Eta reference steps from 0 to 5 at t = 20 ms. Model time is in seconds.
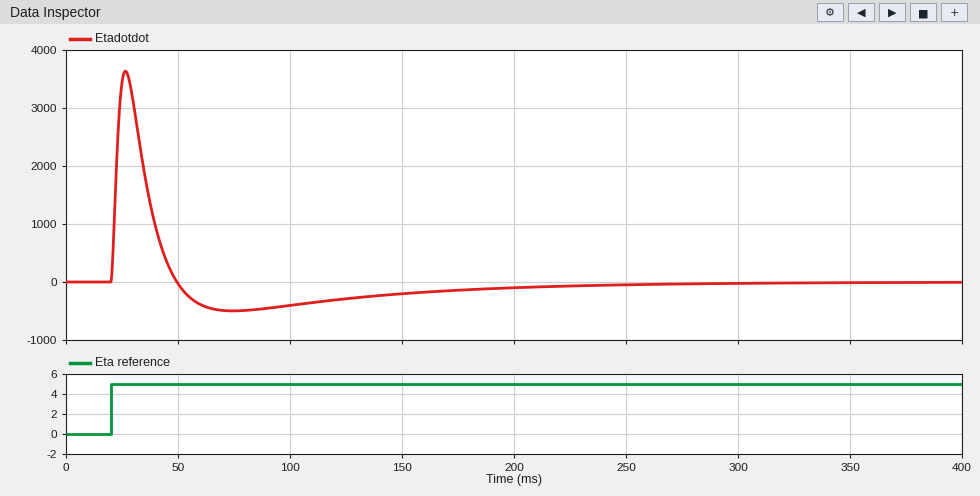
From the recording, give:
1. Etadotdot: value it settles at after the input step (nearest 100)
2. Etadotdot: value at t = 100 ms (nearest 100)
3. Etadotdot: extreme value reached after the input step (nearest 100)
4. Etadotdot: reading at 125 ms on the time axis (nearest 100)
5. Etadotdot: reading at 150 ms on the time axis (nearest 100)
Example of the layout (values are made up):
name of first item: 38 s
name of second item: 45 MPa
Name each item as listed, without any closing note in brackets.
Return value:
Etadotdot: value it settles at after the input step: 0
Etadotdot: value at t = 100 ms: -400
Etadotdot: extreme value reached after the input step: 3600
Etadotdot: reading at 125 ms on the time axis: -300
Etadotdot: reading at 150 ms on the time axis: -200
